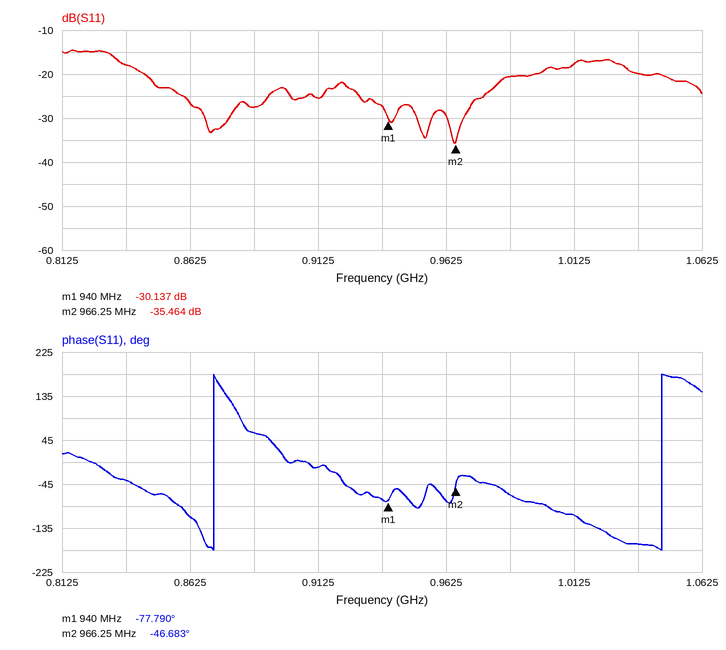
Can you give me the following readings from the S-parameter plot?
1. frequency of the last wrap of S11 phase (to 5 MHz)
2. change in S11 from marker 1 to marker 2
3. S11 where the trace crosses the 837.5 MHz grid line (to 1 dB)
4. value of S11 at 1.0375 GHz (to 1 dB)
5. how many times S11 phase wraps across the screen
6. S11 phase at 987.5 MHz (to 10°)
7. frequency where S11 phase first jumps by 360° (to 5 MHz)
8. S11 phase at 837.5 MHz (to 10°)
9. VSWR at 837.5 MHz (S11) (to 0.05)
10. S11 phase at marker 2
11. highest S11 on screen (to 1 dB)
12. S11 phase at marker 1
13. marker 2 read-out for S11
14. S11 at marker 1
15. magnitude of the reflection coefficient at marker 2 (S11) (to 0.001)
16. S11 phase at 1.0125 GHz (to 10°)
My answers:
1.045 GHz
-5.327 dB
-18 dB
-20 dB
2
-70°
870 MHz
-40°
1.30
-46.683°
-15 dB
-77.790°
-35.464 dB
-30.137 dB
0.017
-110°
